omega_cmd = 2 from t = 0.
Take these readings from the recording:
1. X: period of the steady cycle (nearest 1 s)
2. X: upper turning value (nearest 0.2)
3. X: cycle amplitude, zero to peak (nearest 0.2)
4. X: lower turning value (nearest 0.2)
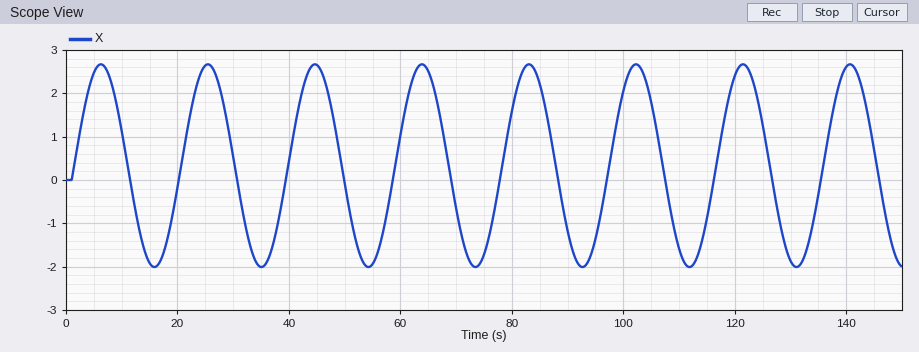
19 s
2.6
2.4
-2.0
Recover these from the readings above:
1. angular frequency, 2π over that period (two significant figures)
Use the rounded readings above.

0.33 rad/s
